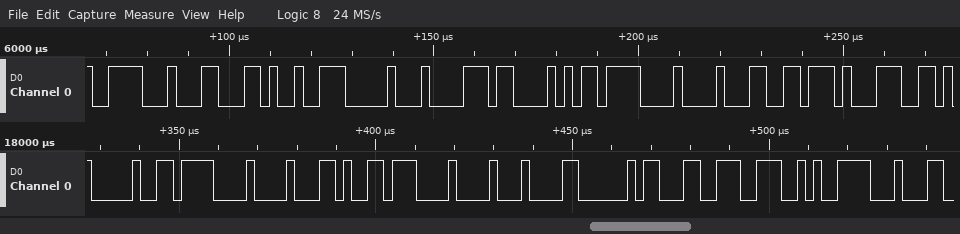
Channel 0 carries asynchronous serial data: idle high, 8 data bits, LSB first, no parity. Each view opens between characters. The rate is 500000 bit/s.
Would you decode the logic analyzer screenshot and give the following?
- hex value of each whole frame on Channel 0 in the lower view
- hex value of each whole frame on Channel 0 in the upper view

90, 0F, 88, D9, 08, 84, A0, CC, 4E, 1E
1E, 8C, C9, 10, B8, A8, 0F, 88, 76, 9C
